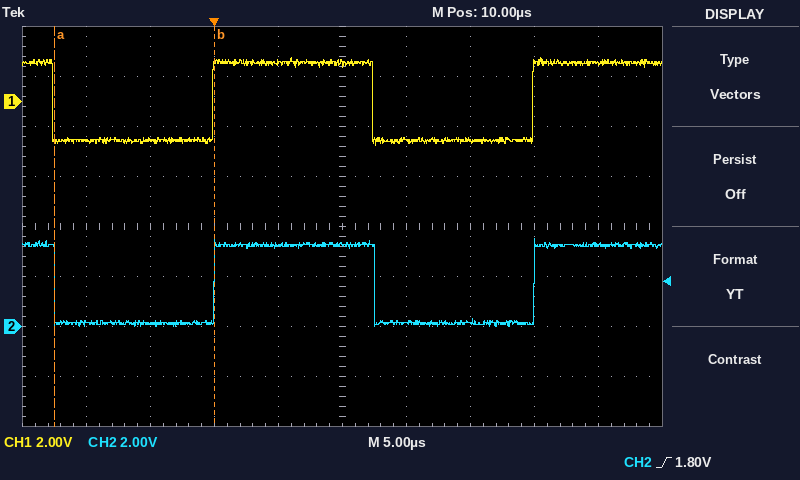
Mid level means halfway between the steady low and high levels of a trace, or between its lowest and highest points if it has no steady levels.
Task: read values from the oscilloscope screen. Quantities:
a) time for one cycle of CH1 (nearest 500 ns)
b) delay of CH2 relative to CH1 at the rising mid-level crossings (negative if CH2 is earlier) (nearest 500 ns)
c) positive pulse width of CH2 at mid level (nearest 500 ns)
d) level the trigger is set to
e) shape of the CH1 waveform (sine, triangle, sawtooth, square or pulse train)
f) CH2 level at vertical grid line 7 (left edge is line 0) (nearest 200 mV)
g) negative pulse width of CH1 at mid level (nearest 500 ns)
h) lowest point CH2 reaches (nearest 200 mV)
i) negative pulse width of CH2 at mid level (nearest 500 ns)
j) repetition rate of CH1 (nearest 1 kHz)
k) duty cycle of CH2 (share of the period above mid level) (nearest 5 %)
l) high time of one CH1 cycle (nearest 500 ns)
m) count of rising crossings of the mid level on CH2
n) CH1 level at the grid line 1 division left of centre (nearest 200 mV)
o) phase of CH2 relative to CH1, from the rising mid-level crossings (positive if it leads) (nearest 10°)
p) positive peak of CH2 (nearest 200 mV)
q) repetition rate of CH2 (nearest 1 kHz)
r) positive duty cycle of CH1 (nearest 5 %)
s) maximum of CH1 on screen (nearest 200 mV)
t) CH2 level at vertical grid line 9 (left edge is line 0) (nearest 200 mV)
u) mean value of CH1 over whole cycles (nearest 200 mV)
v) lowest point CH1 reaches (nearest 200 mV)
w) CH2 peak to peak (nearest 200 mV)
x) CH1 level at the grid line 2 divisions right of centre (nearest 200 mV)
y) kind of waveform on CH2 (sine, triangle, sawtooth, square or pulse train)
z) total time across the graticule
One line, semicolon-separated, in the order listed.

25.0 µs; 0.0 µs; 12.5 µs; 1.80 V; square; 200 mV; 12.5 µs; 0.0 V; 12.5 µs; 40 kHz; 50 %; 12.5 µs; 2; 1.6 V; 0°; 3.6 V; 40 kHz; 50 %; 1.8 V; 3.2 V; 0.0 V; -1.8 V; 3.6 V; -1.6 V; square; 50 µs
